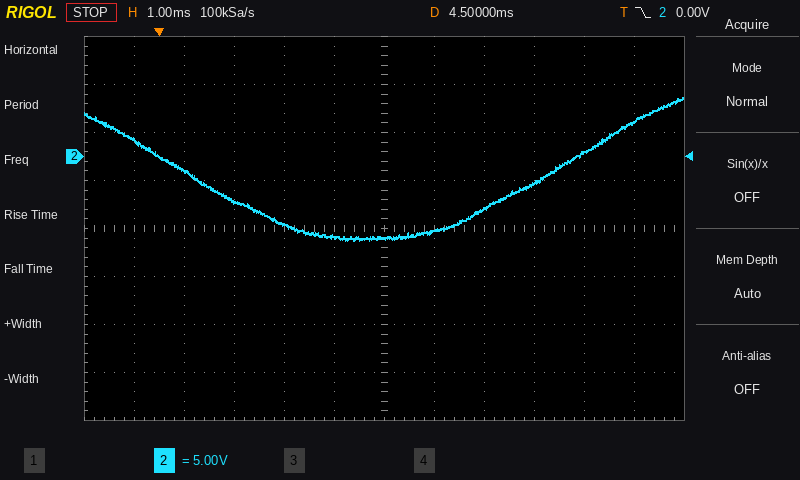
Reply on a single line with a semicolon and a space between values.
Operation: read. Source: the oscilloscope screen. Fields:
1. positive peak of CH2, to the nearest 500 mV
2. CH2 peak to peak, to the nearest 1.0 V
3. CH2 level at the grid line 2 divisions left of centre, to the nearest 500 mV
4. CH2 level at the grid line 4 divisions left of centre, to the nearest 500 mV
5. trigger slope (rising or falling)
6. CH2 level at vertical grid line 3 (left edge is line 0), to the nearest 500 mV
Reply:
6.0 V; 15.0 V; -7.0 V; -1.5 V; falling; -4.5 V
